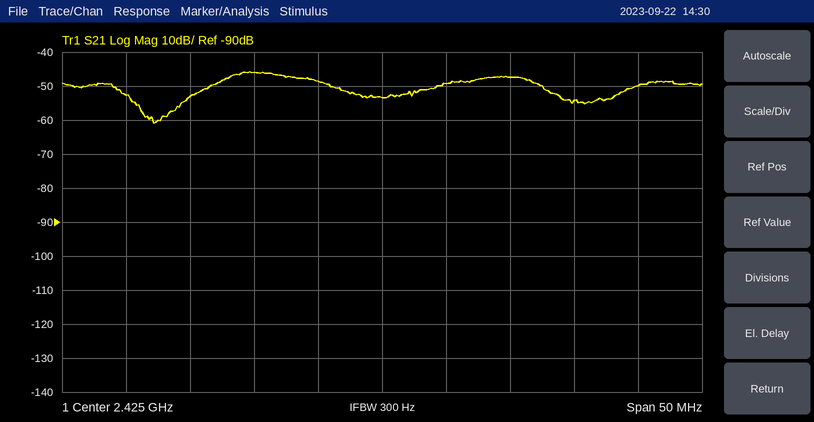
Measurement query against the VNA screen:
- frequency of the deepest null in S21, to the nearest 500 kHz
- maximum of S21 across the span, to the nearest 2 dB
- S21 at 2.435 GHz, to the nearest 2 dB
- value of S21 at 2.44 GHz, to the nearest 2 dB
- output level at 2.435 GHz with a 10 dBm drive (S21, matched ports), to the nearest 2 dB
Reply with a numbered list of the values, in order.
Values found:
1. 2.4070 GHz
2. -46 dB
3. -48 dB
4. -54 dB
5. -38 dBm
